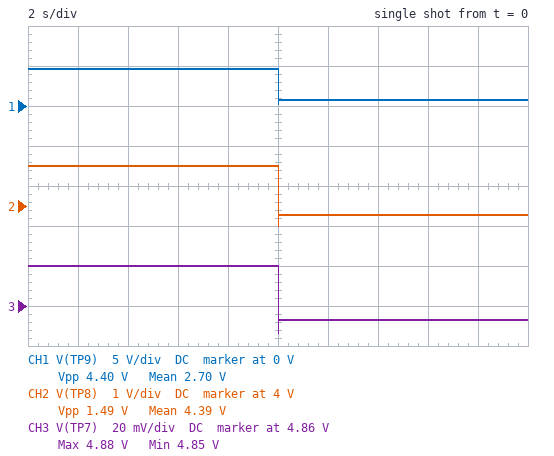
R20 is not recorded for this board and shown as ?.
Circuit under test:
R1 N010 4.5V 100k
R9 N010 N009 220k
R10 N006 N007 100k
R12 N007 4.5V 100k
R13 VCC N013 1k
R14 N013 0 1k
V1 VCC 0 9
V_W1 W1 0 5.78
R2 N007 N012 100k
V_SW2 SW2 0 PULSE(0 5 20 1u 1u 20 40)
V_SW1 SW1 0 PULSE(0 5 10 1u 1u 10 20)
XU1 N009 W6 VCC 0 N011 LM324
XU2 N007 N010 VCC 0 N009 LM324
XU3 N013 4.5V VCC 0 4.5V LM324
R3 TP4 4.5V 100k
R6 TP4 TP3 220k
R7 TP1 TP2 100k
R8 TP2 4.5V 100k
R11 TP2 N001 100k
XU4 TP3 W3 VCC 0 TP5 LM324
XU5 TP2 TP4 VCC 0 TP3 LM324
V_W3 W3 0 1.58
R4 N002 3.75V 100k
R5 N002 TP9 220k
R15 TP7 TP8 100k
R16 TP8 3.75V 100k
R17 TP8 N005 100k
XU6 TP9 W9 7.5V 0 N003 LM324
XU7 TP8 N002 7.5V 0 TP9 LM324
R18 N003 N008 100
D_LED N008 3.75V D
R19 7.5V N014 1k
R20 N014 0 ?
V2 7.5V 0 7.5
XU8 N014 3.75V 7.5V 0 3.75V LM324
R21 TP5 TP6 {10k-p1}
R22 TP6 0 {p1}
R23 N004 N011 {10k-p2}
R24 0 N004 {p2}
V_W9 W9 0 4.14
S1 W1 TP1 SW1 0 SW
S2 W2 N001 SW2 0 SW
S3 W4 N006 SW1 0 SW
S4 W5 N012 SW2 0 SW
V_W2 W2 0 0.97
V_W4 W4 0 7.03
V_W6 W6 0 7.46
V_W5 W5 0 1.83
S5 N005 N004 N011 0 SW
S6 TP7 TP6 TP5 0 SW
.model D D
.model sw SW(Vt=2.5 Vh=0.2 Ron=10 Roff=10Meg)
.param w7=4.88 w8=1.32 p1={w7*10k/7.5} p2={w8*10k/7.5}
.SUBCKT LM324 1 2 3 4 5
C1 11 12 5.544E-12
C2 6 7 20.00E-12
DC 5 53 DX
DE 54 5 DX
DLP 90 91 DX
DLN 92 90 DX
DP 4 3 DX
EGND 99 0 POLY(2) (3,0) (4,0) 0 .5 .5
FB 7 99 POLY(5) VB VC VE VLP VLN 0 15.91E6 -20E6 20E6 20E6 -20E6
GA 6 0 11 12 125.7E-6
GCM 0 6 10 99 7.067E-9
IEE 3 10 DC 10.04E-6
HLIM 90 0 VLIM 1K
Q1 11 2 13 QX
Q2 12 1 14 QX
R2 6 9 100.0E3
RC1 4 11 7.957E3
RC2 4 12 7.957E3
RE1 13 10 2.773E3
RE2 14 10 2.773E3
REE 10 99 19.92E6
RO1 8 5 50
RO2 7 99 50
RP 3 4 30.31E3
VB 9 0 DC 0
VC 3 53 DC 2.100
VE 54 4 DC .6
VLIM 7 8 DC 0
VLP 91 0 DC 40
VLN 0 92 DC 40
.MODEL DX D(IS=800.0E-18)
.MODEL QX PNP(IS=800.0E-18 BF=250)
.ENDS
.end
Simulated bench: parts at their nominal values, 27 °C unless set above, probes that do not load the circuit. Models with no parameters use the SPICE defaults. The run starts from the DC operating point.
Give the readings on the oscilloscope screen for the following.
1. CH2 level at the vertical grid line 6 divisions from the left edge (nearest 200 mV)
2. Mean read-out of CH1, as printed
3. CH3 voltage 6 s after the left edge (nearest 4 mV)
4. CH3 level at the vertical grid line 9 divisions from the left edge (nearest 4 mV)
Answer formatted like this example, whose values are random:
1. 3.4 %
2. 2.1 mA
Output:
1. 3.8 V
2. 2.70 V
3. 4.880 V
4. 4.852 V
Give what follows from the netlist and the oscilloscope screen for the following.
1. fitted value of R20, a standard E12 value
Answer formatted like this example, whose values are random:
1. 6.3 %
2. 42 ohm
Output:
1. 2.2 kΩ
